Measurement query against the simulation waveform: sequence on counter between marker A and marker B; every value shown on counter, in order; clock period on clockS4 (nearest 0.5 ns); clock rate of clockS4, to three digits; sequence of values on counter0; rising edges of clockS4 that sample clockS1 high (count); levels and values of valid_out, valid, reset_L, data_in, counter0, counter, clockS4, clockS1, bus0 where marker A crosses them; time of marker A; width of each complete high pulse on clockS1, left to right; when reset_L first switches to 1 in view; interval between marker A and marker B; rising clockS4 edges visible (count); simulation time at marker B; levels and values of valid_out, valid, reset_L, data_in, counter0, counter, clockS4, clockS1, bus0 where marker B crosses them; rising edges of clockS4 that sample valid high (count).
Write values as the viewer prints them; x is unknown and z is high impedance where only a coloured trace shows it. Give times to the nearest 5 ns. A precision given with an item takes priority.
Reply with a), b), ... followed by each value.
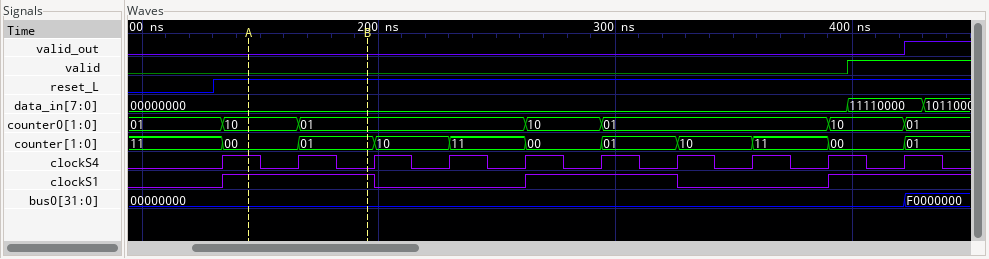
a) 00, 01
b) 11, 00, 01, 10, 11, 00, 01, 10, 11, 00, 01
c) 32 ns
d) 31.2 MHz
e) 01, 10, 01, 10, 01, 10, 01
f) 5
g) valid_out=0, valid=0, reset_L=1, data_in=00000000, counter0=10, counter=00, clockS4=1, clockS1=1, bus0=00000000
h) 145 ns
i) 65 ns, 65 ns
j) 130 ns
k) 50 ns
l) 10
m) 195 ns
n) valid_out=0, valid=0, reset_L=1, data_in=00000000, counter0=01, counter=01, clockS4=0, clockS1=1, bus0=00000000
o) 1
